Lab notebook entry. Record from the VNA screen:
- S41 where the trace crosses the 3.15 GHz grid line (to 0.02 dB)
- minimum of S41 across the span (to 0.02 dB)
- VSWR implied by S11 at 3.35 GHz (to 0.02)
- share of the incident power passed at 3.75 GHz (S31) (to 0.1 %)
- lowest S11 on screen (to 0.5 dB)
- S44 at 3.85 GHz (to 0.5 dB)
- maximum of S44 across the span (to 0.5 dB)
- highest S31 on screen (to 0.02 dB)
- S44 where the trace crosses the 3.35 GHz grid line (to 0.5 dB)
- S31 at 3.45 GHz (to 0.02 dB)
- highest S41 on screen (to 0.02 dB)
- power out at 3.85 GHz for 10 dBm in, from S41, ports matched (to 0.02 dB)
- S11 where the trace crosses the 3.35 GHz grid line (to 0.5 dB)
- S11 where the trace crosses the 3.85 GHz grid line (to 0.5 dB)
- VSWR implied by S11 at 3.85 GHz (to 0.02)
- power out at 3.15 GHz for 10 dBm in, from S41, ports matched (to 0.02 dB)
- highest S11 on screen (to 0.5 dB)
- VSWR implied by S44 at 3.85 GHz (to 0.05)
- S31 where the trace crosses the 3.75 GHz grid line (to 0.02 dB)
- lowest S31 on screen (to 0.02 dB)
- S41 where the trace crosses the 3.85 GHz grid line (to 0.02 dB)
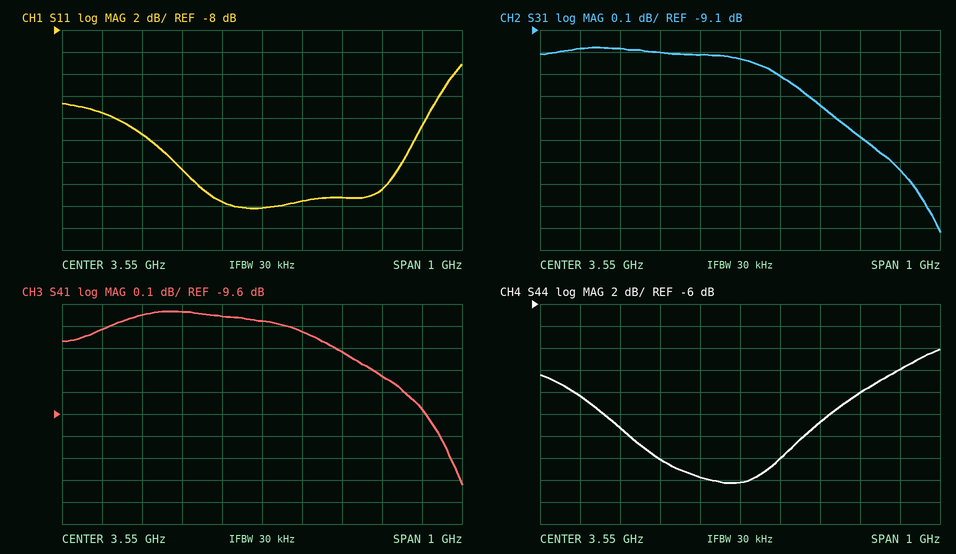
-9.22 dB
-9.92 dB
1.20
11.4 %
-24.0 dB
-14.0 dB
-10.0 dB
-9.18 dB
-20.0 dB
-9.22 dB
-9.14 dB
0.58 dBm
-20.5 dB
-22.5 dB
1.16
0.78 dBm
-11.0 dB
1.50
-9.44 dB
-10.02 dB
-9.42 dB
